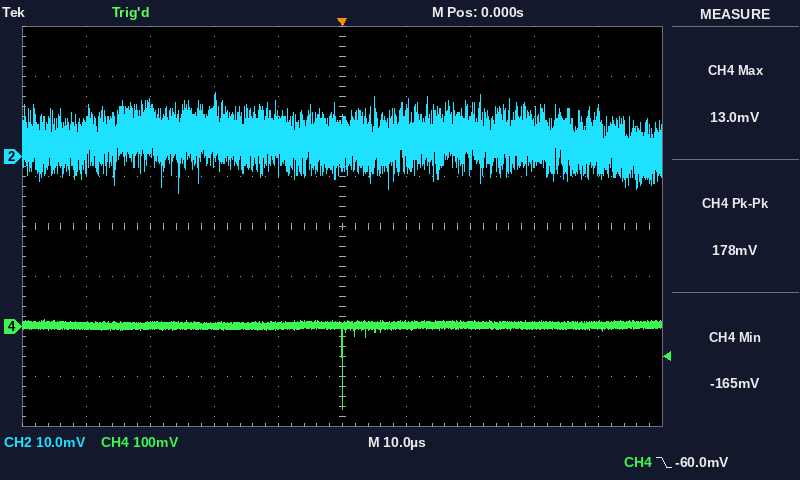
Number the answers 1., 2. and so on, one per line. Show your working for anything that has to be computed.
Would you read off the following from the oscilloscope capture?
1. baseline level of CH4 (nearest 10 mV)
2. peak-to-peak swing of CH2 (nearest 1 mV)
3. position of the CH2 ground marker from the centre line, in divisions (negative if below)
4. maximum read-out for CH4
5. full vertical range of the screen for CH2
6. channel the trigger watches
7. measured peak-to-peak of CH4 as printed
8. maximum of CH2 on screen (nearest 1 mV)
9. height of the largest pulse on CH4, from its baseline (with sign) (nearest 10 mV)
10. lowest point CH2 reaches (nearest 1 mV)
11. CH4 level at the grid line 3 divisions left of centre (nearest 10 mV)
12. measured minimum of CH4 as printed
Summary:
1. 0 mV
2. 13 mV − (-7 mV) = 20 mV
3. +1.4 div
4. 13.0 mV
5. 80 mV
6. CH4
7. 178 mV
8. 13 mV
9. -170 mV
10. -7 mV
11. 0 mV
12. -165 mV
